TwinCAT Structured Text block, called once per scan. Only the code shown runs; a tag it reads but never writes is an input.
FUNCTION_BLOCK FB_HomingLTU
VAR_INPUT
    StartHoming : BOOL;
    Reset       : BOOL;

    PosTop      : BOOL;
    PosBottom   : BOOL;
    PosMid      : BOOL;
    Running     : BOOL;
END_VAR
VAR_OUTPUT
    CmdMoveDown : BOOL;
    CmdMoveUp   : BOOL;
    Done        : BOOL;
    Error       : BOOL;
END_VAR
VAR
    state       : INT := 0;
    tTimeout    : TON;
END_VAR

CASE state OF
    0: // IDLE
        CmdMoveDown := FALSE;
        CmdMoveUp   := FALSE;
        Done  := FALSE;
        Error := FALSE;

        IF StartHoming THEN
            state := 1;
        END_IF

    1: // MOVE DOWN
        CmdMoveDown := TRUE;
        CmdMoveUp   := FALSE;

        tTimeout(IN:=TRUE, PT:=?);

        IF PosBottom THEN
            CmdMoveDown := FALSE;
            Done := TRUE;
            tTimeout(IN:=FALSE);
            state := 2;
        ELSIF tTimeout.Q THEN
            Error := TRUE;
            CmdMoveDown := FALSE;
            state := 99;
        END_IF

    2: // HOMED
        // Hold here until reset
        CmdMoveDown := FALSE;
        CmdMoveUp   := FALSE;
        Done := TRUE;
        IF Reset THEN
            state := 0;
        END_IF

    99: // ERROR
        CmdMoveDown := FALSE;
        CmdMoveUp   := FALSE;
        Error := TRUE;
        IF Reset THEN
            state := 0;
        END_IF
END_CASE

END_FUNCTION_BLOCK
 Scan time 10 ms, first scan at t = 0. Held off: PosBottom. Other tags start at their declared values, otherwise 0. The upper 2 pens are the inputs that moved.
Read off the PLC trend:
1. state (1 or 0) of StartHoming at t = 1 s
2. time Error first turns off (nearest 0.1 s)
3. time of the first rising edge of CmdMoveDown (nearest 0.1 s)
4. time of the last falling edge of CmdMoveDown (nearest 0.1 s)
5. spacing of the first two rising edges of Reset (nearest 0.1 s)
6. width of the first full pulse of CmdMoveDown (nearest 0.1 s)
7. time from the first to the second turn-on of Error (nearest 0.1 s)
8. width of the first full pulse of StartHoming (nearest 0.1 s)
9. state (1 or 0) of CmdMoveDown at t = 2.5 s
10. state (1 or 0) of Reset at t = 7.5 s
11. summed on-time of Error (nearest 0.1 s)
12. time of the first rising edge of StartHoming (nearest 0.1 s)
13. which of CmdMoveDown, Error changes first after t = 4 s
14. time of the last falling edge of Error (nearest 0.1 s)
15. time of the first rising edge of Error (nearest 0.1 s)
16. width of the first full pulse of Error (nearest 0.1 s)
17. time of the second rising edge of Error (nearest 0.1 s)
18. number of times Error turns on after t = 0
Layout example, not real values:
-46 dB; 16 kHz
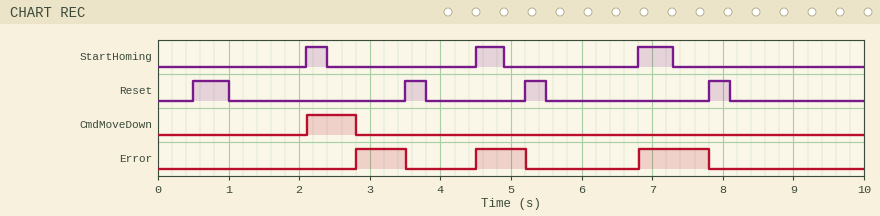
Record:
0; 3.5 s; 2.1 s; 2.8 s; 3.0 s; 0.7 s; 1.7 s; 0.3 s; 1; 0; 2.4 s; 2.1 s; Error; 7.8 s; 2.8 s; 0.7 s; 4.5 s; 3
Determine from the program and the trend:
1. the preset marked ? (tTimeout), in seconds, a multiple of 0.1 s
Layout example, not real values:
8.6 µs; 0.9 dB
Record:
0.7 s
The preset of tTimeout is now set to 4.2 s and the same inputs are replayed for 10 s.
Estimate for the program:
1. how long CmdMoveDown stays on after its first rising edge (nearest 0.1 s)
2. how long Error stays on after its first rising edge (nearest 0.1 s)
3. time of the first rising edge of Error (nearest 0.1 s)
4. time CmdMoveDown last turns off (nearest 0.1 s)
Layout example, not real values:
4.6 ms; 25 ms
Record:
4.2 s; 1.5 s; 6.3 s; 6.3 s
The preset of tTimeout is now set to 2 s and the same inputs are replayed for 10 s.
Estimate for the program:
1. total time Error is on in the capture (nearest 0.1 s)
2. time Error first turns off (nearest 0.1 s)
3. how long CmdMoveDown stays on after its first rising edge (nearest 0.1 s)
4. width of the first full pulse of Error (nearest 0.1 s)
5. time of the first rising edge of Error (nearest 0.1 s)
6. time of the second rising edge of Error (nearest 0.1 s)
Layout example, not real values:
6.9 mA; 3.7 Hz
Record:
2.1 s; 5.2 s; 2.0 s; 1.1 s; 4.1 s; 6.8 s
